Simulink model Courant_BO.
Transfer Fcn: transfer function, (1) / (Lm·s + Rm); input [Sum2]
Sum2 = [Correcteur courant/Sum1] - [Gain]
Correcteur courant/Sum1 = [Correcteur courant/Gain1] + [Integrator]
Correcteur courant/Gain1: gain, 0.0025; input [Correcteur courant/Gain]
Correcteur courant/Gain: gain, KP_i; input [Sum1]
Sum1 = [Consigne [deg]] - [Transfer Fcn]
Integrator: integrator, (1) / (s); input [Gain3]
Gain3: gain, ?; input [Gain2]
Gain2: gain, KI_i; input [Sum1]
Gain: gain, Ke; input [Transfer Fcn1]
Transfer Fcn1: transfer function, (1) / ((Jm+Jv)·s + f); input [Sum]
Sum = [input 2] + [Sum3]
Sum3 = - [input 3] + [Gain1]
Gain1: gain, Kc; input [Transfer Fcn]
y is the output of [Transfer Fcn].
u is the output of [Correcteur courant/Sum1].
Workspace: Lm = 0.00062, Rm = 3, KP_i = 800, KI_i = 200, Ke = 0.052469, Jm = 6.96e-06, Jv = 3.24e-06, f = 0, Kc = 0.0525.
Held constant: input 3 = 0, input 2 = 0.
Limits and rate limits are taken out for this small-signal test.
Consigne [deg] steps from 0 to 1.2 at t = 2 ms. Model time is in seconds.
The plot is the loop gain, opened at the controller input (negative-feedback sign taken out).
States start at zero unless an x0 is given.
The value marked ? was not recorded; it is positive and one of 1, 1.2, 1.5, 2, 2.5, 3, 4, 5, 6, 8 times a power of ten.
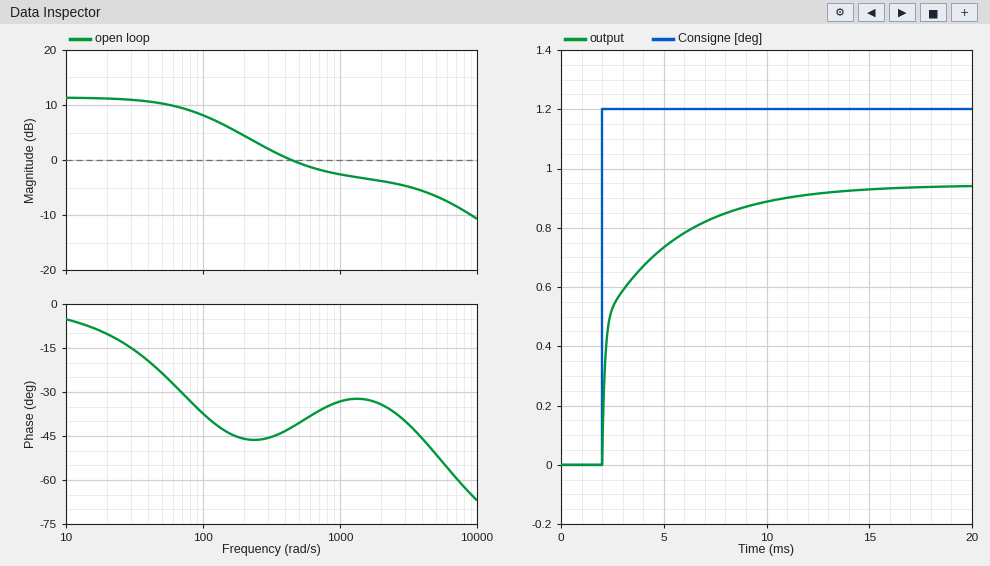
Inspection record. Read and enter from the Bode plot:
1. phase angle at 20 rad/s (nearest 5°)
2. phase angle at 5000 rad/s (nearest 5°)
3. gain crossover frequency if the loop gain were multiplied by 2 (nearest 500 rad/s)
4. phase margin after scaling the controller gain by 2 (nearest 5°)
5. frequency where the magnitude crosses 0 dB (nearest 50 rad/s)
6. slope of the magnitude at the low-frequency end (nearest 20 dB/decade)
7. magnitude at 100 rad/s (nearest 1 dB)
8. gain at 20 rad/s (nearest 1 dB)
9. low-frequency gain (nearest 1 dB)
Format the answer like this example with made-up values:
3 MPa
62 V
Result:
-10°
-50°
4500 rad/s
130°
450 rad/s
0 dB/decade
8 dB
11 dB
11 dB
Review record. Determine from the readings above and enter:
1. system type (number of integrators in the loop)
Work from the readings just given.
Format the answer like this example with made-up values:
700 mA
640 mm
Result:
0
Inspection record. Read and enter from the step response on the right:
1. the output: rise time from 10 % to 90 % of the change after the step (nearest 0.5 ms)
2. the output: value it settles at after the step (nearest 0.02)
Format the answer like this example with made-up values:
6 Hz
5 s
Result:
6.0 ms
0.94
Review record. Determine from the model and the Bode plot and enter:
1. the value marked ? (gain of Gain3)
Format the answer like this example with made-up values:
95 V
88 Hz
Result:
5
